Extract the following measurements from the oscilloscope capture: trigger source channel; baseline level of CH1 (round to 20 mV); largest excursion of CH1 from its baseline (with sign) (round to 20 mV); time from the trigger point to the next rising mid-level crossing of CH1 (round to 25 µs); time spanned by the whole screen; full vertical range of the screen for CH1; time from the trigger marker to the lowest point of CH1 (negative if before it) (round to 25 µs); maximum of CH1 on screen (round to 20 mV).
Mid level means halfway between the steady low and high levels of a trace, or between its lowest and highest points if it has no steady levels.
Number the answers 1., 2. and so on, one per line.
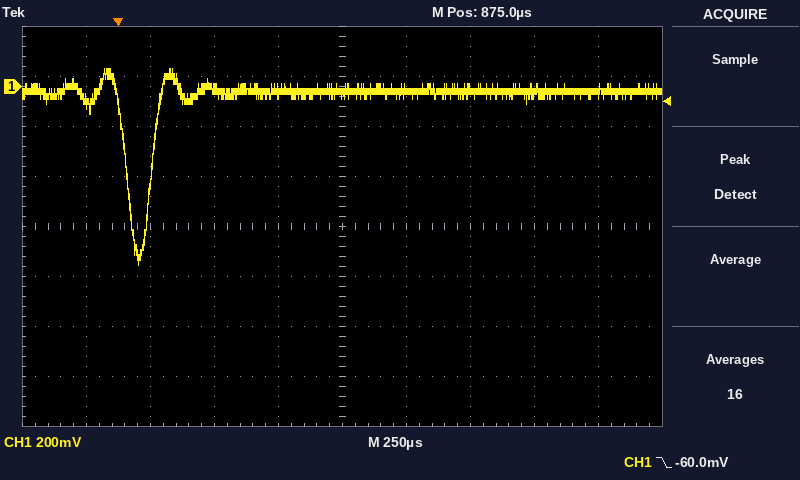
1. CH1
2. -20 mV
3. -700 mV
4. 125 µs
5. 2.5 ms
6. 1.6 V
7. +75 µs
8. 80 mV
